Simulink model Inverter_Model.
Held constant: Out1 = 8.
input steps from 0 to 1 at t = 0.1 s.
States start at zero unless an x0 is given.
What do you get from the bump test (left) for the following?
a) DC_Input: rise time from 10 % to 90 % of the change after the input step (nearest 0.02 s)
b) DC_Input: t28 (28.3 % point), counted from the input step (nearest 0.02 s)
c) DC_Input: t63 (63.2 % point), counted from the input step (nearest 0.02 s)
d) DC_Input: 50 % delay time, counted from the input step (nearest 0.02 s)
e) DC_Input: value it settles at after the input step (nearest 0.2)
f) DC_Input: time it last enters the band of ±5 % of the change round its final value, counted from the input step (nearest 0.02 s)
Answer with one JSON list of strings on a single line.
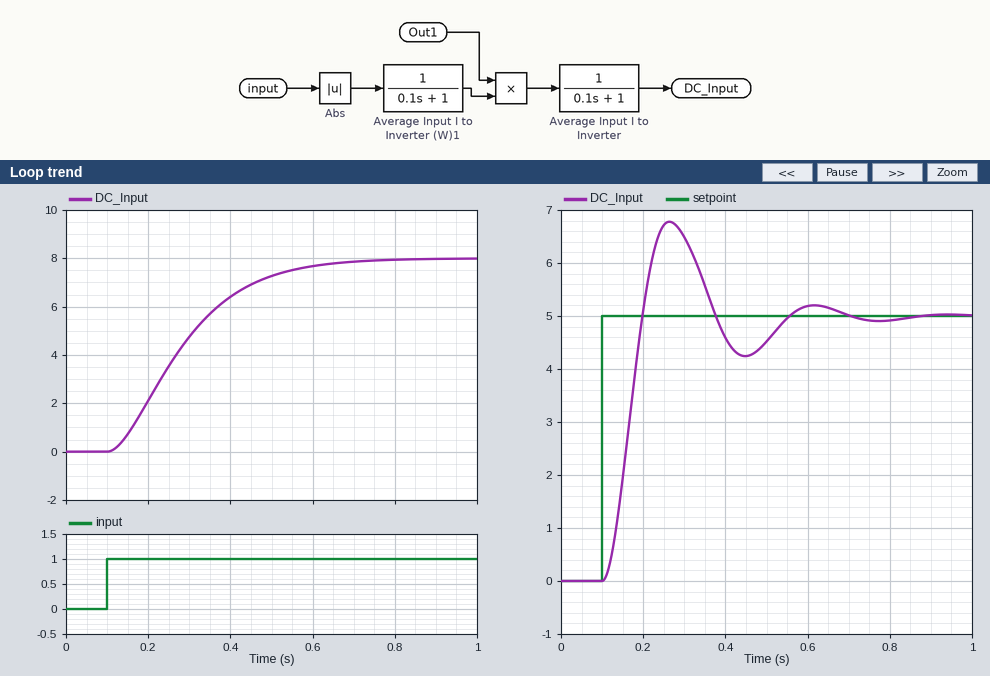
["0.34 s", "0.10 s", "0.22 s", "0.16 s", "8.0", "0.48 s"]
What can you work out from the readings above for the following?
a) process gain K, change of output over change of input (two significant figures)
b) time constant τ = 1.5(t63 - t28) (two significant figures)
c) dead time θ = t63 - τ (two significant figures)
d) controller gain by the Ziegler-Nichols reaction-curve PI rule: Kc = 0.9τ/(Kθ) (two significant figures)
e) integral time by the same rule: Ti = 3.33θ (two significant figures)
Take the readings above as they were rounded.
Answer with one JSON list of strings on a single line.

["8.0", "0.18 s", "0.040 s", "0.51", "0.13 s"]
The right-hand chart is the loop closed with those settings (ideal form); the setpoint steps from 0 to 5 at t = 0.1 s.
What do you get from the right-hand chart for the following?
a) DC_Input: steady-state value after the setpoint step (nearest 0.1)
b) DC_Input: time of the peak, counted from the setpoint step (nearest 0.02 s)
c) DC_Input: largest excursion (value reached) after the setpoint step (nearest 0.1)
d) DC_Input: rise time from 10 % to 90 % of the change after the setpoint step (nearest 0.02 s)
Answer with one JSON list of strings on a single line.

["5.0", "0.16 s", "6.8", "0.06 s"]
